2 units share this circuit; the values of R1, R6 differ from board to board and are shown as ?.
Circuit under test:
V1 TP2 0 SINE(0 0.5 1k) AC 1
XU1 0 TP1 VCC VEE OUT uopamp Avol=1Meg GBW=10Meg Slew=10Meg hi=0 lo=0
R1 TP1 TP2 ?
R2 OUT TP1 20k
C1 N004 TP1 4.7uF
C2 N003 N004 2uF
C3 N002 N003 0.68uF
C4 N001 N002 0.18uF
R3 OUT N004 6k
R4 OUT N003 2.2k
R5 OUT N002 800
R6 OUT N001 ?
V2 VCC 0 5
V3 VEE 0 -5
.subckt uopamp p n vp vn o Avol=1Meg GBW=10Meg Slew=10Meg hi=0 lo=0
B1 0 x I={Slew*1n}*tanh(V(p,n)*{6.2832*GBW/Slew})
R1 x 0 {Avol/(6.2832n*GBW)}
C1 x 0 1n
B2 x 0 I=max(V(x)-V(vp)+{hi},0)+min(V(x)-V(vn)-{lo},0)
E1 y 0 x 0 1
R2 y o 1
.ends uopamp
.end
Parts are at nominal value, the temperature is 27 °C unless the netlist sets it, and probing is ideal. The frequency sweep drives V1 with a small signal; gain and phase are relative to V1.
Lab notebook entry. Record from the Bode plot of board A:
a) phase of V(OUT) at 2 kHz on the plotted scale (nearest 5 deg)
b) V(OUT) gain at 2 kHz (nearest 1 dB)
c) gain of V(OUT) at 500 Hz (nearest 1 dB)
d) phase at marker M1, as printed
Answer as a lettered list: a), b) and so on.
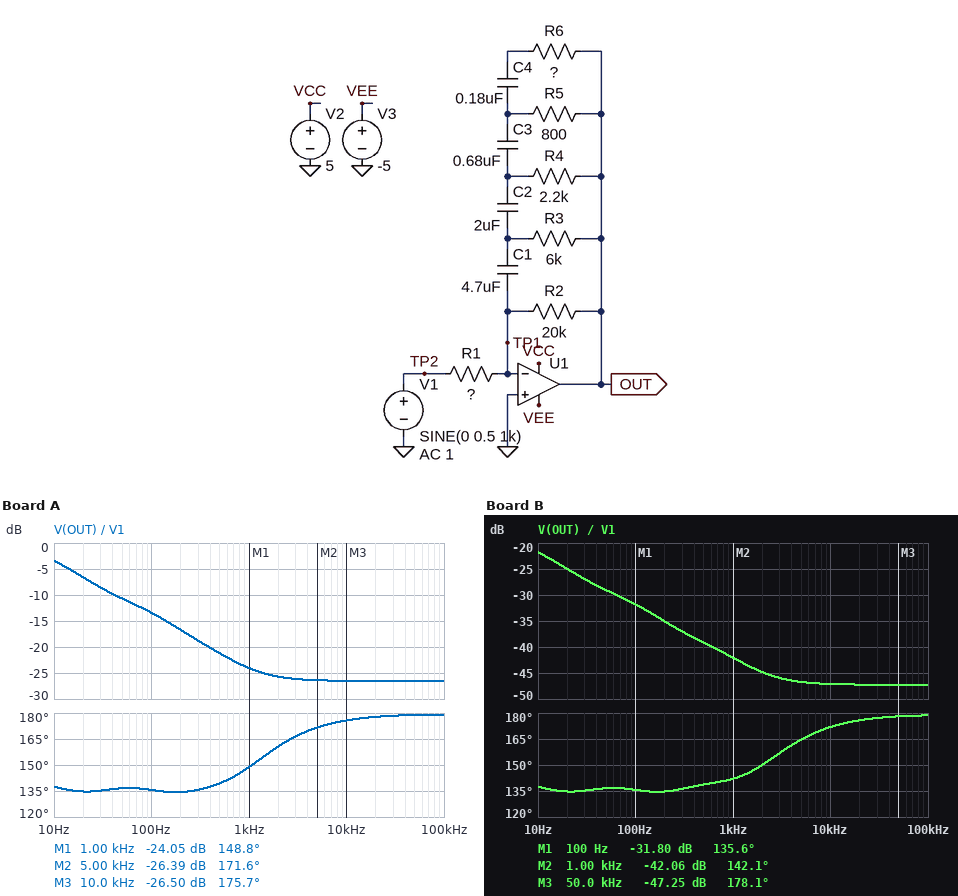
a) 160 deg
b) -26 dB
c) -21 dB
d) 148.8 deg
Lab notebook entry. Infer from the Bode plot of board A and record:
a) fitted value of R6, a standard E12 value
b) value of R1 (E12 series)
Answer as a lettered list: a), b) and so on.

a) 1.5 kΩ
b) 8.2 kΩ
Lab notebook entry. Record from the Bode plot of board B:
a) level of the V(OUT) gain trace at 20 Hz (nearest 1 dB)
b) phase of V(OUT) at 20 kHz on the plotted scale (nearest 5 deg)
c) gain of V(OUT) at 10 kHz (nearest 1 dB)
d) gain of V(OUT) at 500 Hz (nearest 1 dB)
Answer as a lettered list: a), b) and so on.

a) -25 dB
b) 175 deg
c) -47 dB
d) -39 dB
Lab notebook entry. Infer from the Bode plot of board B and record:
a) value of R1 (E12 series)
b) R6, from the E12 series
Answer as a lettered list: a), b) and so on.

a) 68 kΩ
b) 680 Ω
